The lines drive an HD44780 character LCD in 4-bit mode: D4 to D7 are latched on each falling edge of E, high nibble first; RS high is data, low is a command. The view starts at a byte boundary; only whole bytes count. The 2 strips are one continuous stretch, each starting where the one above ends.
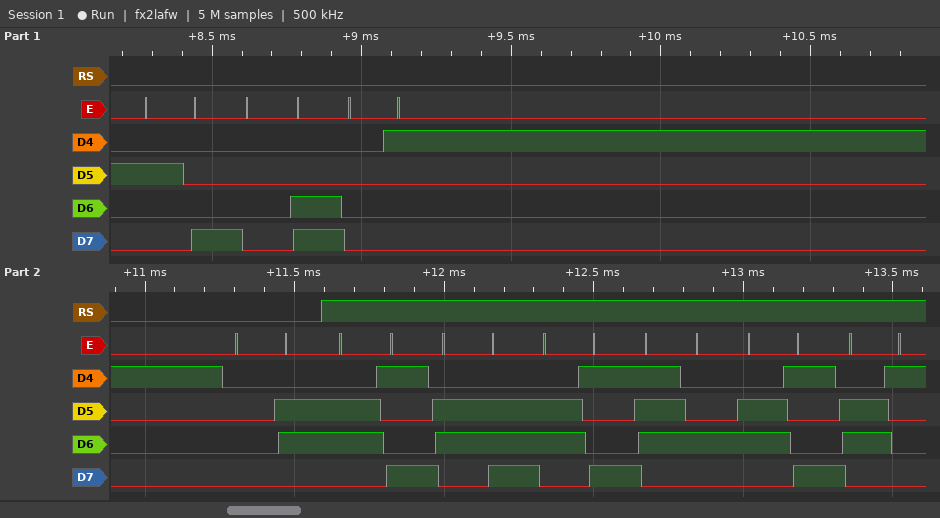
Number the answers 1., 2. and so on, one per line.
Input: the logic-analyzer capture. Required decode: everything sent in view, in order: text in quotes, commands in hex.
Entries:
1. 0x28 0x0C 0x01 0x06 "initia"
